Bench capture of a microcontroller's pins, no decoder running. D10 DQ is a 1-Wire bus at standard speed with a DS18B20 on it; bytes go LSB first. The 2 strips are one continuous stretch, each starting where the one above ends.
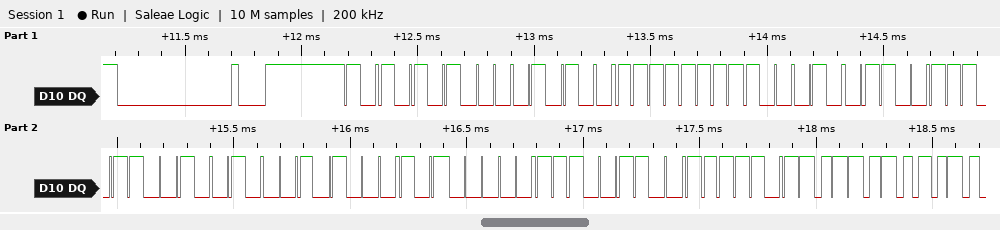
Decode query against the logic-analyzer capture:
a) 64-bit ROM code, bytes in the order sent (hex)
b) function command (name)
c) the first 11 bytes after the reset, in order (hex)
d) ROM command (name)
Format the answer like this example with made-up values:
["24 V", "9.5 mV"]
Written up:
["28 FF 91 B9 49 14 05 67", "Read Scratchpad", "55 28 FF 91 B9 49 14 05 67 BE 2D", "Match ROM"]
